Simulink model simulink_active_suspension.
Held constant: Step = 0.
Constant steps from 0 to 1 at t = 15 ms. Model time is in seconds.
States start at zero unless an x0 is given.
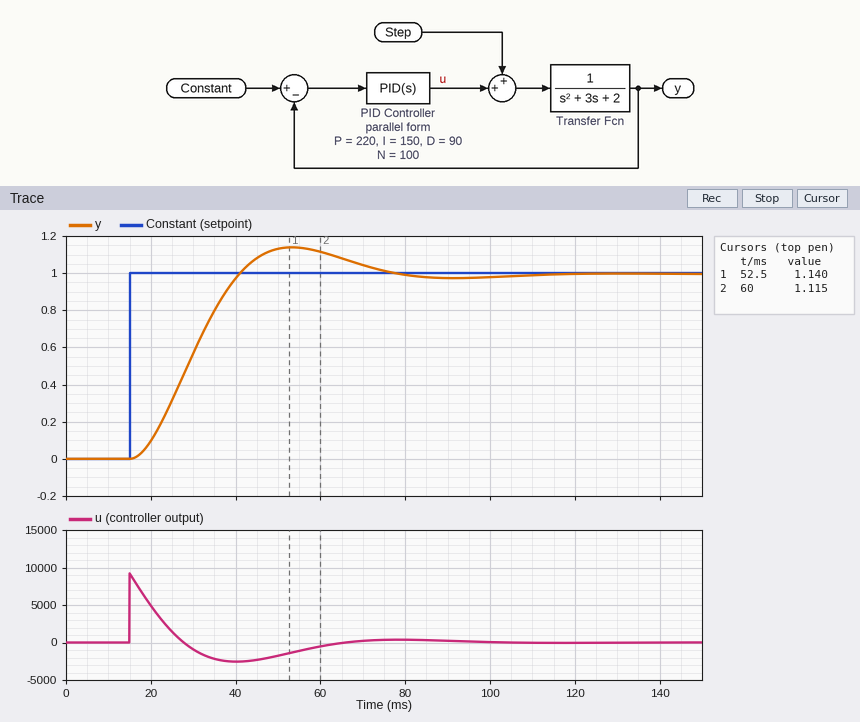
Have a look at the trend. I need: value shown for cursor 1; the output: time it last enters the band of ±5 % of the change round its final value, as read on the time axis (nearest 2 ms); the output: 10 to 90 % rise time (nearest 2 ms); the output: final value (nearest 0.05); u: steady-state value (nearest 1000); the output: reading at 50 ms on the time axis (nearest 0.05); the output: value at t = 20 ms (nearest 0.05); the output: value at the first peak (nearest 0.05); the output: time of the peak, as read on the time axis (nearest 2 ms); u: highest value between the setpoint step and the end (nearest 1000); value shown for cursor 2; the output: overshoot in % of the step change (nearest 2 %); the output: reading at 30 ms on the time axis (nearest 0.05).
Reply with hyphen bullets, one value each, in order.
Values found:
- 1.140
- 70 ms
- 18 ms
- 1.00
- 0
- 1.15
- 0.10
- 1.15
- 54 ms
- 9000
- 1.115
- 14 %
- 0.55
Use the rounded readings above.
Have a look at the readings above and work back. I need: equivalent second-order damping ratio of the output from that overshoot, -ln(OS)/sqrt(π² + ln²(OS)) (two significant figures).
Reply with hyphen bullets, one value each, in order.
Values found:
- 0.53
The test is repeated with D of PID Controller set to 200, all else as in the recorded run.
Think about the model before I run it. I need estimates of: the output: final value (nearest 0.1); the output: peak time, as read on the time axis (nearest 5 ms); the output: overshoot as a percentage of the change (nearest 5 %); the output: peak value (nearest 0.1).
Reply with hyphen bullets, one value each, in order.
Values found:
- 1.0
- 40 ms
- 30 %
- 1.3
